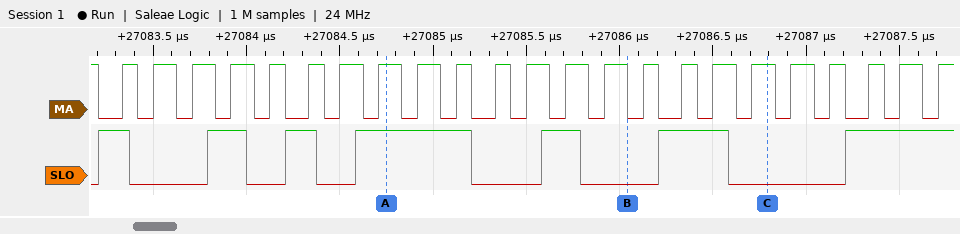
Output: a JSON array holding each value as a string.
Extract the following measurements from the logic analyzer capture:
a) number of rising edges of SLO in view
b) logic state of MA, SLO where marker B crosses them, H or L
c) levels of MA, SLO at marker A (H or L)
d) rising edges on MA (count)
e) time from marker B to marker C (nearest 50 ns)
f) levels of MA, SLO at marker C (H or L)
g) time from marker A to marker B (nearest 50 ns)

["7", "MA=L, SLO=L", "MA=H, SLO=H", "23", "750 ns", "MA=H, SLO=L", "1300 ns"]
